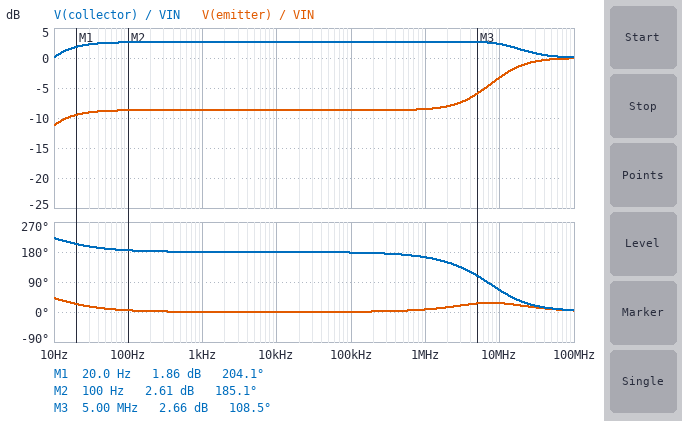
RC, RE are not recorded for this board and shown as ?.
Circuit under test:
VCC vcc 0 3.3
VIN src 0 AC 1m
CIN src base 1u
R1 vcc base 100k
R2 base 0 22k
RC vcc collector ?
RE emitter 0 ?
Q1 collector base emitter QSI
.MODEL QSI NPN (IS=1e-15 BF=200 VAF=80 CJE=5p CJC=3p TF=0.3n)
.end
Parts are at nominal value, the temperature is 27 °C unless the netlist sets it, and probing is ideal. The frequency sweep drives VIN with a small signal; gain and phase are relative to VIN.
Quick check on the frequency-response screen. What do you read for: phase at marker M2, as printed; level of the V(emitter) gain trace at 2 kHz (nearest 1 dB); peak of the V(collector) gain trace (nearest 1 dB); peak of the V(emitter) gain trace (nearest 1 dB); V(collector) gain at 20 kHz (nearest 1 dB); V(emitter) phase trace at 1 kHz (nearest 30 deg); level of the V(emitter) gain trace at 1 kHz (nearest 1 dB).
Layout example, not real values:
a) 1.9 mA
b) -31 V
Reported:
a) 185.1 deg
b) -9 dB
c) 3 dB
d) 0 dB
e) 3 dB
f) 0 deg
g) -9 dB
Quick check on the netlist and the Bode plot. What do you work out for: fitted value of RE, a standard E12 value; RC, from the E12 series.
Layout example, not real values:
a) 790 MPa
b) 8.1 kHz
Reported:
a) 2.7 kΩ
b) 10 kΩ
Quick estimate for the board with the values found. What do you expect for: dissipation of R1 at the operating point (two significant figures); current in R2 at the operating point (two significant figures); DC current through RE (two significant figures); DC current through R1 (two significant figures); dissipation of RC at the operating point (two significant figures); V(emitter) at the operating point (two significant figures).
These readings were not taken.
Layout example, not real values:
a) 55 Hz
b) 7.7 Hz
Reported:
a) 73 µW
b) 27 µA
c) 5.6 µA
d) 27 µA
e) 310 nW
f) 15 mV
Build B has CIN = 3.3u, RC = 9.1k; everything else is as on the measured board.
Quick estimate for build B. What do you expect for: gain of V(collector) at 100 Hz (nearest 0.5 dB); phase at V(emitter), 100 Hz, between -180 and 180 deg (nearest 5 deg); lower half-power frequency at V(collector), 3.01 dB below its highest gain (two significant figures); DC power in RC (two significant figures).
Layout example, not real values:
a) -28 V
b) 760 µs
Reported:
a) 2.0 dB
b) 0 deg
c) 2.9 Hz
d) 280 nW
